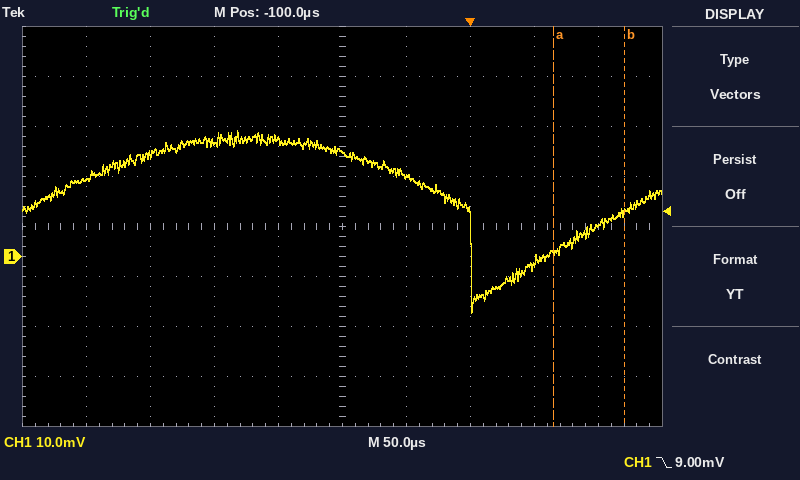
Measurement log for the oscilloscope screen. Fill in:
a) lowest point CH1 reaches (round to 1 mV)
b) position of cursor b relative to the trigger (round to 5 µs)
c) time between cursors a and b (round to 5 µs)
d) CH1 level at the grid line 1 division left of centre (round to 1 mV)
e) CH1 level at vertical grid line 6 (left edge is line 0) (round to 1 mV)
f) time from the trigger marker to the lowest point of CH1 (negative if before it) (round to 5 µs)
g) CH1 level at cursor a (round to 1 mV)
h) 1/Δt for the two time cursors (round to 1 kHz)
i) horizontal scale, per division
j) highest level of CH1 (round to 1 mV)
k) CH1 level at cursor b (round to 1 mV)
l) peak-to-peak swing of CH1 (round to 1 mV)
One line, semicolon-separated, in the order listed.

-11 mV; +120 µs; 55 µs; 23 mV; 16 mV; 0 µs; 1 mV; 18 kHz; 50 µs; 25 mV; 9 mV; 36 mV
